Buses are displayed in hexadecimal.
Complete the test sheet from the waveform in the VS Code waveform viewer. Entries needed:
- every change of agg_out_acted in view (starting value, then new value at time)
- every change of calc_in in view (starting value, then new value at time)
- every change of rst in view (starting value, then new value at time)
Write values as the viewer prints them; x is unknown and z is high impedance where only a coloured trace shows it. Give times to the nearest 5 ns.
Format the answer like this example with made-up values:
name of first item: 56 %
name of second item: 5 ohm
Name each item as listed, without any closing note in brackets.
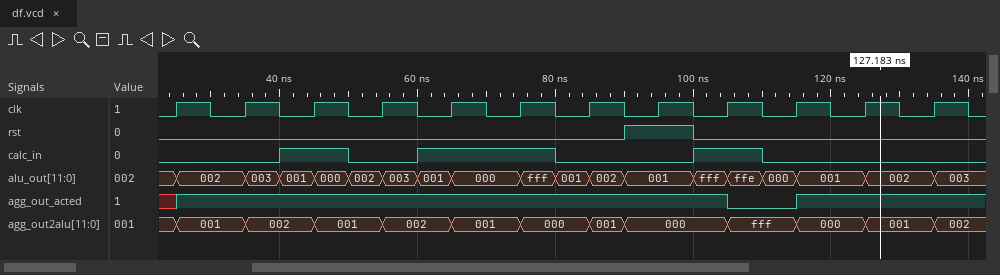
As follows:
every change of agg_out_acted in view: x, 1 at 25 ns, 0 at 105 ns, 1 at 115 ns
every change of calc_in in view: 0, 1 at 40 ns, 0 at 50 ns, 1 at 60 ns, 0 at 80 ns, 1 at 100 ns, 0 at 110 ns
every change of rst in view: 0, 1 at 90 ns, 0 at 100 ns
